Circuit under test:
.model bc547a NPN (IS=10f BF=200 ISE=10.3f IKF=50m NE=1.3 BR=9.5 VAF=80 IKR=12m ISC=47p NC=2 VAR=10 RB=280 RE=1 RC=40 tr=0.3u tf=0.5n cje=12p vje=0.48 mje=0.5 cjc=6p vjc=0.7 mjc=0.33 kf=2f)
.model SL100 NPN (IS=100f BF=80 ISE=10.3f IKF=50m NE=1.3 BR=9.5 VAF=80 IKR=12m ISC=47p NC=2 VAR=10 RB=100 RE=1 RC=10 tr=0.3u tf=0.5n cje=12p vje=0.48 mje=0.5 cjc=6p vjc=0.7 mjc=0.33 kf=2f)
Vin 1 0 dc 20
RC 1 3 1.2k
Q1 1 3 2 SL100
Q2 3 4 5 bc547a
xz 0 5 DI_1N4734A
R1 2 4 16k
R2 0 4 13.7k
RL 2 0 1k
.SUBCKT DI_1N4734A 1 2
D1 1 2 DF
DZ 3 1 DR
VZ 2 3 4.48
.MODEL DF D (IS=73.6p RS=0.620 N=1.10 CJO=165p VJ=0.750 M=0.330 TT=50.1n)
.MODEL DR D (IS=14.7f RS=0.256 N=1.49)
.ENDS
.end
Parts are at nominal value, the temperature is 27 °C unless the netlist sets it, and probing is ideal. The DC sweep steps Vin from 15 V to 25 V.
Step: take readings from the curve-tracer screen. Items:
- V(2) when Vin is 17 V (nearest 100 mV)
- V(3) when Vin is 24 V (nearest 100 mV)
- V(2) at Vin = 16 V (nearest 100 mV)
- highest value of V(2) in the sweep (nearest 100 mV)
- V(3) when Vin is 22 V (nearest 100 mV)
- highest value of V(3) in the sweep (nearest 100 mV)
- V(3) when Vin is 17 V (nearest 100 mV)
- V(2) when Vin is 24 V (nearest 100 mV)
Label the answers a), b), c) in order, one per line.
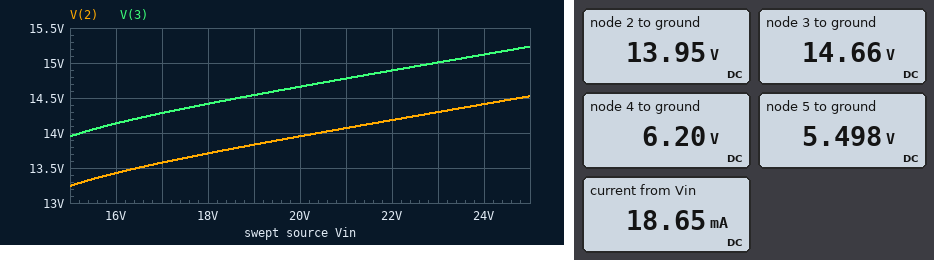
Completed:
a) 13.6 V
b) 15.1 V
c) 13.4 V
d) 14.5 V
e) 14.9 V
f) 15.2 V
g) 14.3 V
h) 14.4 V
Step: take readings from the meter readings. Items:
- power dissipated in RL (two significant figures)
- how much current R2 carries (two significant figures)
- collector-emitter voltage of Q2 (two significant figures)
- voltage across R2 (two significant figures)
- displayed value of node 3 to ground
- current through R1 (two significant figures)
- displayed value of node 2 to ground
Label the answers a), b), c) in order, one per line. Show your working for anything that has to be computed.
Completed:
a) (13.95 V)^2 / 1 kΩ = 190 mW
b) (6.2 V) / 13.7 kΩ = 450 µA
c) 14.66 V - 5.498 V = 9.2 V
d) 6.2 V = 6.2 V
e) 14.66 V
f) (13.95 V - 6.2 V) / 16 kΩ = 480 µA
g) 13.95 V
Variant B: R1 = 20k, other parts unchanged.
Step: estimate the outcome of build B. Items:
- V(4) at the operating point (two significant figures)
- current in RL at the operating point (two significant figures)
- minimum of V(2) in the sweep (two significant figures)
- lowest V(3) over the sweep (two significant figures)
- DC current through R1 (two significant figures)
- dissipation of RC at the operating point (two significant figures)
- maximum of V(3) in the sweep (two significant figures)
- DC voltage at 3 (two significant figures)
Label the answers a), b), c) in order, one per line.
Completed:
a) 6.2 V
b) 16 mA
c) 14 V
d) 15 V
e) 470 µA
f) 11 mW
g) 17 V
h) 16 V
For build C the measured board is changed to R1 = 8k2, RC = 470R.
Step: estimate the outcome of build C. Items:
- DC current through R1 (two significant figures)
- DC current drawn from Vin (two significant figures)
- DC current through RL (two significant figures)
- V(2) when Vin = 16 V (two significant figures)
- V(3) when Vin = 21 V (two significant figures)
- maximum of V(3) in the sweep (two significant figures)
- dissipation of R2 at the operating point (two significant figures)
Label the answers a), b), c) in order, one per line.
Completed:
a) 610 µA
b) 29 mA
c) 11 mA
d) 11 V
e) 12 V
f) 13 V
g) 2.9 mW
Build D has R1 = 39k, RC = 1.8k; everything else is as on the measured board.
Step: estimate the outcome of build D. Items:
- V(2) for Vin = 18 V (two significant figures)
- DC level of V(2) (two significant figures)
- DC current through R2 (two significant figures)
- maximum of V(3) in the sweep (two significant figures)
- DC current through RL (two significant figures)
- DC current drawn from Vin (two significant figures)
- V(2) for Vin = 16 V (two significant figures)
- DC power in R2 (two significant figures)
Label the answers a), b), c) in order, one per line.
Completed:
a) 17 V
b) 19 V
c) 350 µA
d) 24 V
e) 19 mA
f) 19 mA
g) 15 V
h) 1.7 mW
